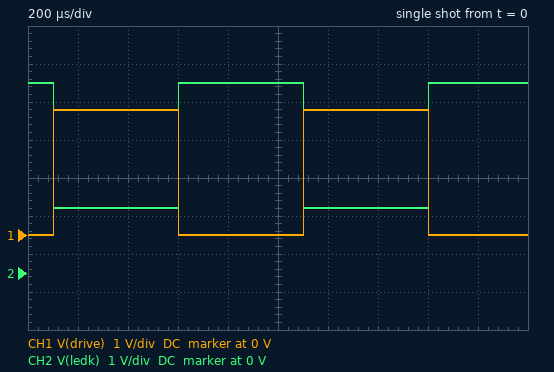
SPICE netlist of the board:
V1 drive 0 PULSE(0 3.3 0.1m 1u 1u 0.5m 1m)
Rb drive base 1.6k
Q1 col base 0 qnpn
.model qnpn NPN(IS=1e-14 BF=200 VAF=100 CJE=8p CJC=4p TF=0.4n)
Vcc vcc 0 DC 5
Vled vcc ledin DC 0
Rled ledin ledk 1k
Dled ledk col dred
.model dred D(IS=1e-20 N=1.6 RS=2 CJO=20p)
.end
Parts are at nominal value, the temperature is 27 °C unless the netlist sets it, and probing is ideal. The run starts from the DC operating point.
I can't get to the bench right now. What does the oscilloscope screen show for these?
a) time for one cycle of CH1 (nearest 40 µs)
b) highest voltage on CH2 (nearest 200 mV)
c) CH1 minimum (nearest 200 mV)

1.00 ms
5.0 V
0 V
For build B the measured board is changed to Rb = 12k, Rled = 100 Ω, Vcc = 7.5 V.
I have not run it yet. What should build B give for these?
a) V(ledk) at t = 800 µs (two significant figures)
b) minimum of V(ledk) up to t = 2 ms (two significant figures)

7.5 V
3.2 V
